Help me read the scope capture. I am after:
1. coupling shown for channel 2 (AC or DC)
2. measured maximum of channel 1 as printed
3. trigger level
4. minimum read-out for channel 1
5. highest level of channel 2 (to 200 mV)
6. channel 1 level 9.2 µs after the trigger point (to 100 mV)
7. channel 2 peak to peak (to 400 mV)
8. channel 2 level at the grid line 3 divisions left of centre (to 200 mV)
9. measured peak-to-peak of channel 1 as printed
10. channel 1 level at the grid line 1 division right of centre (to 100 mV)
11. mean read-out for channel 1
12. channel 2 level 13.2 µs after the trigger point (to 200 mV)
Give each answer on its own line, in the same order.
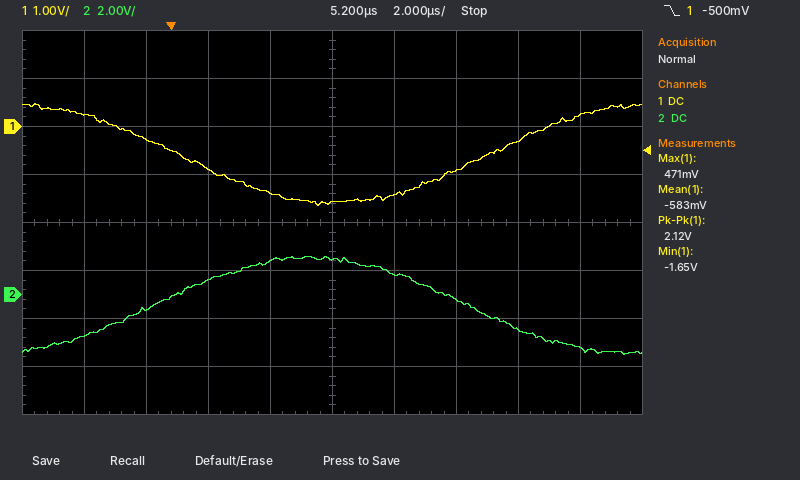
DC
471 mV
-500 mV
-1.65 V
1.6 V
-900 mV
4.0 V
-600 mV
2.12 V
-1.4 V
-583 mV
-2.2 V
